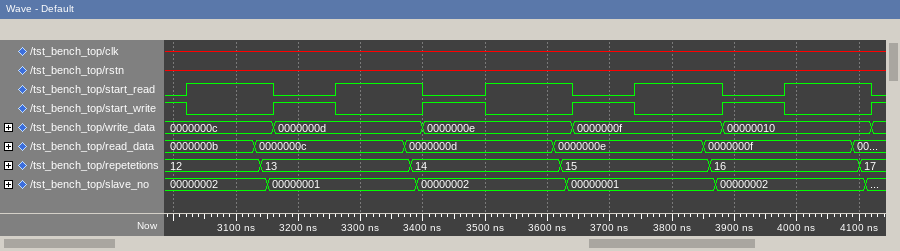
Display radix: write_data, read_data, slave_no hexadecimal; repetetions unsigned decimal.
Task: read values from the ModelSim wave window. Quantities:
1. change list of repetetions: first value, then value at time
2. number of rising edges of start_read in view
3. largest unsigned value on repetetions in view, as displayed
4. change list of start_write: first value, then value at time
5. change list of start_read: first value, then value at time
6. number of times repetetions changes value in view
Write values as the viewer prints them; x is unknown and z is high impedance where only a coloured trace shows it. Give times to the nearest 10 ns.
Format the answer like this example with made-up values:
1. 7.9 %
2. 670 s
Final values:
1. 12, 13 at 3140 ns, 14 at 3380 ns, 15 at 3620 ns, 16 at 3860 ns, 17 at 4100 ns
2. 5
3. 17
4. 1, 0 at 3020 ns, 1 at 3160 ns, 0 at 3260 ns, 1 at 3400 ns, 0 at 3500 ns, 1 at 3640 ns, 0 at 3740 ns, 1 at 3880 ns, 0 at 3980 ns, 1 at 4120 ns
5. 0, 1 at 3020 ns, 0 at 3160 ns, 1 at 3260 ns, 0 at 3400 ns, 1 at 3500 ns, 0 at 3640 ns, 1 at 3740 ns, 0 at 3880 ns, 1 at 3980 ns, 0 at 4120 ns
6. 5
